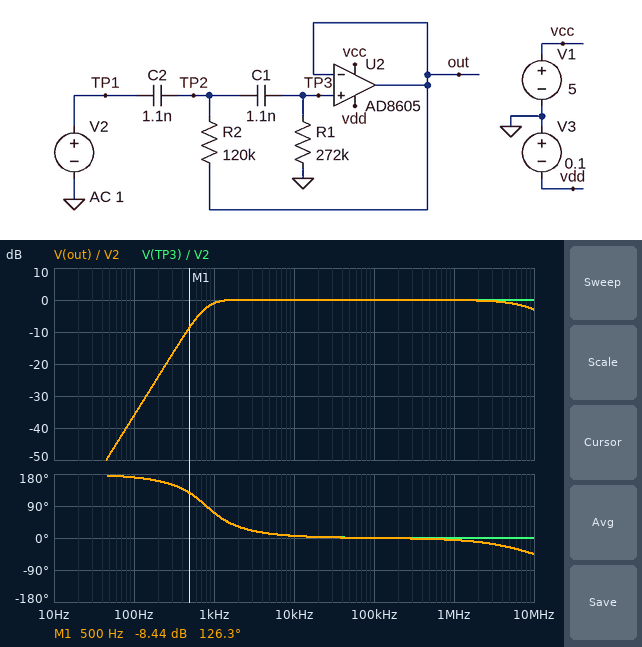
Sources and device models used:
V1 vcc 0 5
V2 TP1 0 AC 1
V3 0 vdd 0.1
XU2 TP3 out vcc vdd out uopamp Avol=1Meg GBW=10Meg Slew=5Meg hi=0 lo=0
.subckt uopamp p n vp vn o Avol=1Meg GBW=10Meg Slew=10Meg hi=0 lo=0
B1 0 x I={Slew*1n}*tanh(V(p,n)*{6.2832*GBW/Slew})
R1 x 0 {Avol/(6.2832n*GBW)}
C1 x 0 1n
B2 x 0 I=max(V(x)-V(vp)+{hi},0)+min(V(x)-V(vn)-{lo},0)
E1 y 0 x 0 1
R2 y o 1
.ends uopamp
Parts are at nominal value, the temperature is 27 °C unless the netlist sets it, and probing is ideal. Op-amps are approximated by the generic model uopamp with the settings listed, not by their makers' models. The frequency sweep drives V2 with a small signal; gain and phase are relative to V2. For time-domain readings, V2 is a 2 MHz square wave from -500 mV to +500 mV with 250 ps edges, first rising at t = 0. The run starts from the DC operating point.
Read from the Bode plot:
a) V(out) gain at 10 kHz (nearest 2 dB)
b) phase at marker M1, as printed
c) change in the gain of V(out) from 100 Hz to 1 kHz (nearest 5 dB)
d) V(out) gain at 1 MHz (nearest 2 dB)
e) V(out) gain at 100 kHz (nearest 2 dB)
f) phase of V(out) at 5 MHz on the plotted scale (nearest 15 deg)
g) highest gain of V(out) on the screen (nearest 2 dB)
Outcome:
0 dB
126.3 deg
35 dB
0 dB
0 dB
-30 deg
0 dB
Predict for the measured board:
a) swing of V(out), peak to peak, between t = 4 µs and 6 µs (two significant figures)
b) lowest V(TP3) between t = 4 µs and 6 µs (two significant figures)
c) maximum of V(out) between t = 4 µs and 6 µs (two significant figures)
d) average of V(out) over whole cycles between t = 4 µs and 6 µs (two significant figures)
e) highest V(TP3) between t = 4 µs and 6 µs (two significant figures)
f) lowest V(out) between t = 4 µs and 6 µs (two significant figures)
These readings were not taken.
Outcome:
1.0 V
-21 mV
980 mV
480 mV
990 mV
-18 mV
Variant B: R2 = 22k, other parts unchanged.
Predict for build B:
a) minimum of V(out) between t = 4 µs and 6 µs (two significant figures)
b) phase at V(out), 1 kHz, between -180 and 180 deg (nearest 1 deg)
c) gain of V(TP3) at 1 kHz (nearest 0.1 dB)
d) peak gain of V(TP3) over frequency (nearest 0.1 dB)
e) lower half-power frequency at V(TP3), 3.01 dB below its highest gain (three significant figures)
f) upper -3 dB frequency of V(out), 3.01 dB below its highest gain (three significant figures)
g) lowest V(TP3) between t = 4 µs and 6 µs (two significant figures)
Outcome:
-19 mV
157 deg
-8.7 dB
5.3 dB
1.59 kHz
3.45 kHz
-25 mV
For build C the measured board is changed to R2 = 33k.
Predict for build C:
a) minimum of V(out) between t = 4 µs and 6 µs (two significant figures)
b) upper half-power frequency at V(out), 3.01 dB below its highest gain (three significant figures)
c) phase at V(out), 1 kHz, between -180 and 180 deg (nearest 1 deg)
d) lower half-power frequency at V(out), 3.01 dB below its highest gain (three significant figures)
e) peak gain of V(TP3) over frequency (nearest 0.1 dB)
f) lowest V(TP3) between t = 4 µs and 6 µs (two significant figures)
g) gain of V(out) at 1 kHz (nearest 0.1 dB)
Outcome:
-19 mV
4.72 kHz
141 deg
1.29 kHz
3.7 dB
-23 mV
-4.6 dB
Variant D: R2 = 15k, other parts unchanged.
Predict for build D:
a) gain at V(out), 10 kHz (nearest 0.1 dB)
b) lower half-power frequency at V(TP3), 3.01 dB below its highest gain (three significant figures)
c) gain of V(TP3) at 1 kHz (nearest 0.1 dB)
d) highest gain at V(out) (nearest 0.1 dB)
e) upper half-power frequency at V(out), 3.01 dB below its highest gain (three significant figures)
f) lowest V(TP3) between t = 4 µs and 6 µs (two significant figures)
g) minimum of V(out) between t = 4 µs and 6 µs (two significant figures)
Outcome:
0.4 dB
1.95 kHz
-12.6 dB
6.8 dB
3.44 kHz
-27 mV
-20 mV
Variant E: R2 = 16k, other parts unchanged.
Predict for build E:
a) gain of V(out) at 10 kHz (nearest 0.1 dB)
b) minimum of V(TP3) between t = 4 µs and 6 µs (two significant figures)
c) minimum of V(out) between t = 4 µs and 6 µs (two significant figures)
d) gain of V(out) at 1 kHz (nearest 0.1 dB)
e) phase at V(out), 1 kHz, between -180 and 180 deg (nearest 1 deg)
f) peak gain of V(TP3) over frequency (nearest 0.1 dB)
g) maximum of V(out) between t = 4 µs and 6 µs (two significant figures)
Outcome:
0.4 dB
-27 mV
-20 mV
-11.9 dB
164 deg
6.5 dB
980 mV
